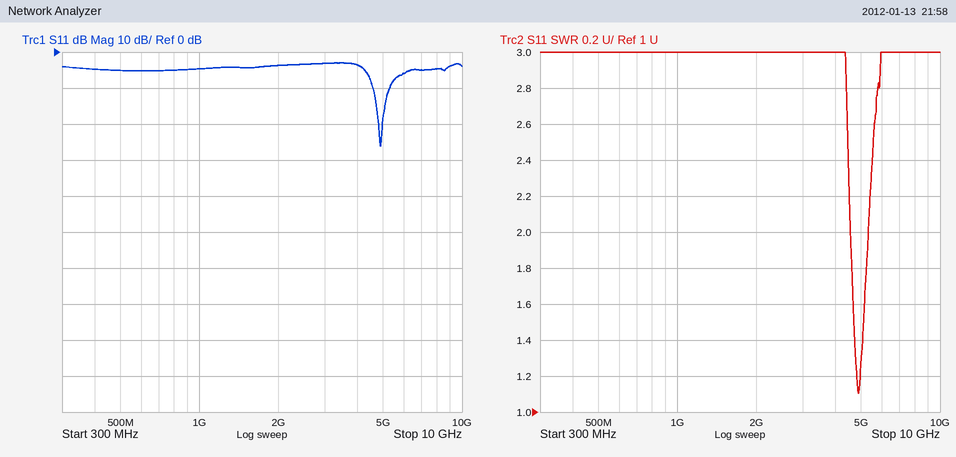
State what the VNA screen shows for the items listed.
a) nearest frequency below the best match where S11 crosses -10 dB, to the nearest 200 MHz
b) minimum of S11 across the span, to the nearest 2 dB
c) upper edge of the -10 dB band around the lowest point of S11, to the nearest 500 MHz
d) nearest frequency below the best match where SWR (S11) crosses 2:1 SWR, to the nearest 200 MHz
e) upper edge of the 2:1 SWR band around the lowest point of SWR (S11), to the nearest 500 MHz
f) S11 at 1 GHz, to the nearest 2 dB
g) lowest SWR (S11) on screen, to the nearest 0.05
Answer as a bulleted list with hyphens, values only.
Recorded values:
- 4.6 GHz
- -26 dB
- 5.5 GHz
- 4.6 GHz
- 5.5 GHz
- -4 dB
- 1.10
